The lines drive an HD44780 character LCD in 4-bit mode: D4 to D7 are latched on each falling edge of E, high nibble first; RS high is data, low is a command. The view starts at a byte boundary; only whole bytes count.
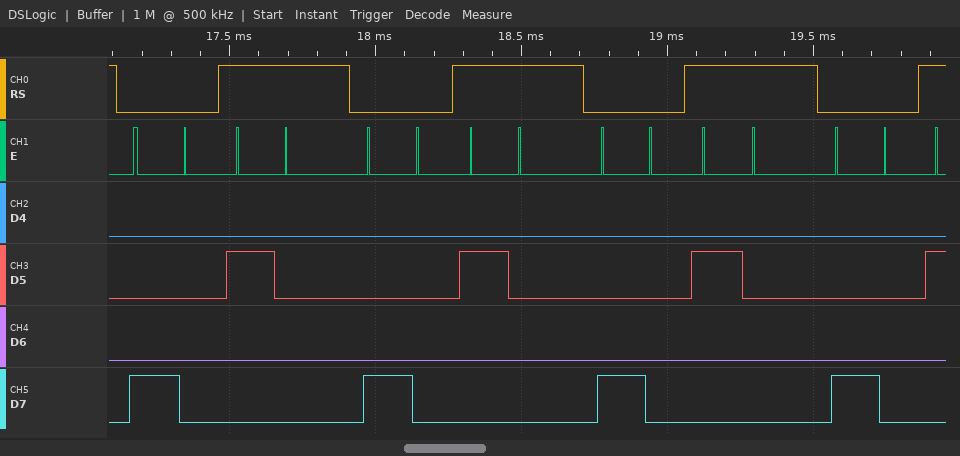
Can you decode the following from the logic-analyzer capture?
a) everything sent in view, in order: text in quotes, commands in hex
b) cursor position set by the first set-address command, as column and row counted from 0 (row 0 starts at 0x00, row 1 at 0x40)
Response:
0x80 " " 0x80 " " 0x80 " " 0x80
column 0, row 0
